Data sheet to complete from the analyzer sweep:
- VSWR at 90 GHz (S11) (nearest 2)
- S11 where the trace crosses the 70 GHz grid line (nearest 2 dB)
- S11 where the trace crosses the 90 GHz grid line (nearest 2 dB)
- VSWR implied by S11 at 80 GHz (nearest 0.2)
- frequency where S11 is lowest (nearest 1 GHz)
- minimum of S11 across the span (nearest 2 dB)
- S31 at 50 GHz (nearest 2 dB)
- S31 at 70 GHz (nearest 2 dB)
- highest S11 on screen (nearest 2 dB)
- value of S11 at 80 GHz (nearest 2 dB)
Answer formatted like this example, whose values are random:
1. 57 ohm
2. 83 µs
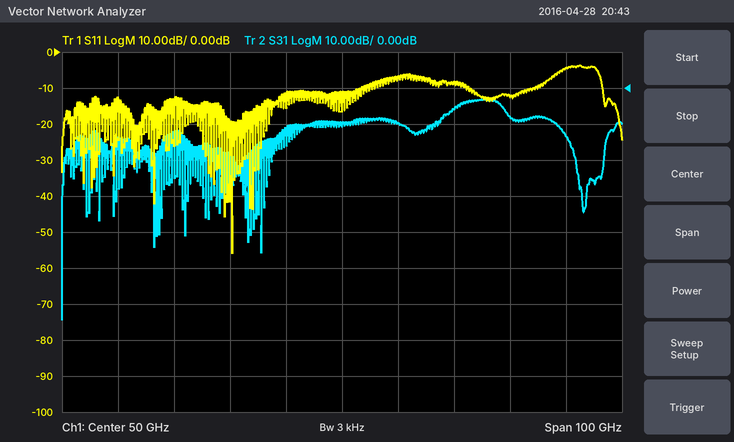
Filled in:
1. 4
2. -8 dB
3. -4 dB
4. 1.6
5. 30 GHz
6. -56 dB
7. -10 dB
8. -6 dB
9. -4 dB
10. -12 dB
